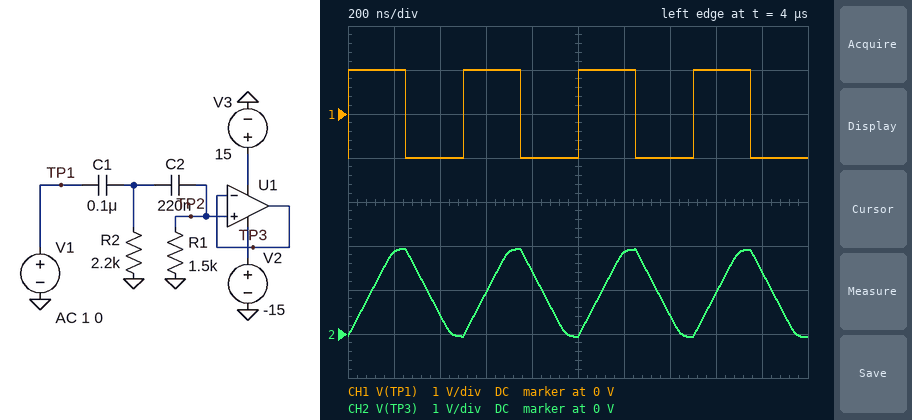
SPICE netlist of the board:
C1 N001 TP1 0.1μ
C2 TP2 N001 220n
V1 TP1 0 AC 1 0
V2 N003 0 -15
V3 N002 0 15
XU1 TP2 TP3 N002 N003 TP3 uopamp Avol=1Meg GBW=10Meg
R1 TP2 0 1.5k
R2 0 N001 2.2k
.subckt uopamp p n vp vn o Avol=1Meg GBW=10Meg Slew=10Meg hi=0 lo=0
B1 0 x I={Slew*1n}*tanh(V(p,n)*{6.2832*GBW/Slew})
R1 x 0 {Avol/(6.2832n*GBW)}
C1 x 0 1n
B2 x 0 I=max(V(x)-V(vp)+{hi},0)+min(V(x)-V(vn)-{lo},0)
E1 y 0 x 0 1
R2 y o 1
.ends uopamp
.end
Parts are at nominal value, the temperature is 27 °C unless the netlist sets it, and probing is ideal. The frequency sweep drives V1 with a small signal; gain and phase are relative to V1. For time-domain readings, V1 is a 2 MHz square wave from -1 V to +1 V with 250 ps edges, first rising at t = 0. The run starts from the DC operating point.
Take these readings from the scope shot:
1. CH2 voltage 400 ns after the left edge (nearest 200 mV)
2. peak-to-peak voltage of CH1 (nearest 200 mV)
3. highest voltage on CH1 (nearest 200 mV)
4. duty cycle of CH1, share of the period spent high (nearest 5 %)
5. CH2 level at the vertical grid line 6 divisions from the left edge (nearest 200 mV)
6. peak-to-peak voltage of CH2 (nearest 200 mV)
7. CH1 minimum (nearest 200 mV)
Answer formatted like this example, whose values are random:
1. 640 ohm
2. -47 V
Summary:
1. 400 mV
2. 2.0 V
3. 1.0 V
4. 50 %
5. 1.8 V
6. 2.0 V
7. -1.0 V
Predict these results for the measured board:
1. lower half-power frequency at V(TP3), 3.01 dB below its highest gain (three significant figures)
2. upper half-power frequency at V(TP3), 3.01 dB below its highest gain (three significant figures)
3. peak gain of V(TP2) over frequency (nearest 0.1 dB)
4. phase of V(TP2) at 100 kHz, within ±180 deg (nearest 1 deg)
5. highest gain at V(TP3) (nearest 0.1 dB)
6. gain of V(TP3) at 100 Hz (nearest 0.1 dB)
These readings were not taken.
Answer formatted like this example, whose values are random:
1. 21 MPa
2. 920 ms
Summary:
1. 2.11 kHz
2. 10.0 MHz
3. 0 dB
4. 1 deg
5. 0 dB
6. -32.2 dB
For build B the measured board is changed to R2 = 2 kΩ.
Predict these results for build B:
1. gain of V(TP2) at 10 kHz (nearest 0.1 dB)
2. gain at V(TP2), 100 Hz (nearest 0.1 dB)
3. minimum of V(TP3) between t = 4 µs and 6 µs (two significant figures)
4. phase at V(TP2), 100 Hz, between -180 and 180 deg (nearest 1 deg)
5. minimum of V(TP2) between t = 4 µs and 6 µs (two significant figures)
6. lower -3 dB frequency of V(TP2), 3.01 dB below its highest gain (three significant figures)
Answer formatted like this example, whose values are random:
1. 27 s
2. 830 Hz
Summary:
1. -0.2 dB
2. -32.9 dB
3. -81 mV
4. 148 deg
5. -85 mV
6. 2.18 kHz
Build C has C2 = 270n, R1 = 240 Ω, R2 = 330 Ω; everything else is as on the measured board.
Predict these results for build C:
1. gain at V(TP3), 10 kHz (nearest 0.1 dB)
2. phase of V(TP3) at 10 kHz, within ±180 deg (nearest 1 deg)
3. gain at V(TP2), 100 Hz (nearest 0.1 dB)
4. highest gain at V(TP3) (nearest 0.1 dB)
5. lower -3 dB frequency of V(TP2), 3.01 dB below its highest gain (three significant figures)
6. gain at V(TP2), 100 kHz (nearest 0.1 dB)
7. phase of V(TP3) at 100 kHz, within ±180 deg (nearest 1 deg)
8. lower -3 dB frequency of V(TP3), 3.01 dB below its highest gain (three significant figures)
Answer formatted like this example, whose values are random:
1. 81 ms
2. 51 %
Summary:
1. -4.3 dB
2. 58 deg
3. -61.5 dB
4. 0 dB
5. 13.1 kHz
6. -0.1 dB
7. 7 deg
8. 13.0 kHz
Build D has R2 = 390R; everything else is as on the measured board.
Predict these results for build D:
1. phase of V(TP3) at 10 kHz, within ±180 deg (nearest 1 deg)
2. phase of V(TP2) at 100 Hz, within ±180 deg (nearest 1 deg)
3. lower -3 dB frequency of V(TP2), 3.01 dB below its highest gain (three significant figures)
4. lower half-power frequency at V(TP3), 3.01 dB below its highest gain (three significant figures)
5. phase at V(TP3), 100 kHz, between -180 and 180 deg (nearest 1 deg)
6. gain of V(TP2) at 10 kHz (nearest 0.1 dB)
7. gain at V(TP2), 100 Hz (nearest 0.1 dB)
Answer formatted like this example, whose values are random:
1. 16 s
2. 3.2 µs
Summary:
1. 30 deg
2. 164 deg
3. 5.28 kHz
4. 5.27 kHz
5. 3 deg
6. -1.1 dB
7. -46.2 dB
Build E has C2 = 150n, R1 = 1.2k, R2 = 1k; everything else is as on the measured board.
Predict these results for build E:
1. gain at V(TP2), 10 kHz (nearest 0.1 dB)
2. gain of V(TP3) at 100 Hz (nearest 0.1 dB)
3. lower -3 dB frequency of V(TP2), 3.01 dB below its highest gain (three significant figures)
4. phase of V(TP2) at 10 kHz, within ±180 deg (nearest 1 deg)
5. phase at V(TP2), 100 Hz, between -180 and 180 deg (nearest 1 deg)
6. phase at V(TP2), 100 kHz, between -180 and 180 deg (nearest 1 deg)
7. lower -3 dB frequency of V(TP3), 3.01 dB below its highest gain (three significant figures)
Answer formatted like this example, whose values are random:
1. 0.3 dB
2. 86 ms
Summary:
1. -0.5 dB
2. -43.2 dB
3. 3.44 kHz
4. 21 deg
5. 165 deg
6. 2 deg
7. 3.43 kHz
